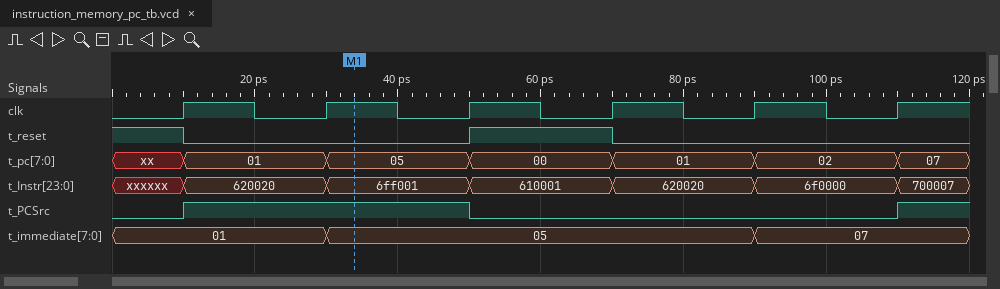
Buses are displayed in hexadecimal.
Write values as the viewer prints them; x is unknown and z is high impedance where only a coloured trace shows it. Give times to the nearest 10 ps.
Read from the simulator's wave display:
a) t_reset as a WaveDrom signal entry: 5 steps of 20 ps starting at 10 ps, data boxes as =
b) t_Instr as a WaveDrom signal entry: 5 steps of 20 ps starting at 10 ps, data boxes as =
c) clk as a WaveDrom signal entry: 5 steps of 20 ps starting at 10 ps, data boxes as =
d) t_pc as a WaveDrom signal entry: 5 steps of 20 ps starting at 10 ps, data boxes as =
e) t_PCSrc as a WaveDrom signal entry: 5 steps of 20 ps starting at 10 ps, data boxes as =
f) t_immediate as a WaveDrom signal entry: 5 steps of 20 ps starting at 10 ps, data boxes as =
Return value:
{name: 't_reset', wave: '0.10.'}
{name: 't_Instr', wave: '=====', data: '620020 6ff001 610001 620020 6f0000'}
{name: 'clk', wave: 'p....'}
{name: 't_pc', wave: '=====', data: '01 05 00 01 02'}
{name: 't_PCSrc', wave: '1.0..'}
{name: 't_immediate', wave: '==..=', data: '01 05 07'}
